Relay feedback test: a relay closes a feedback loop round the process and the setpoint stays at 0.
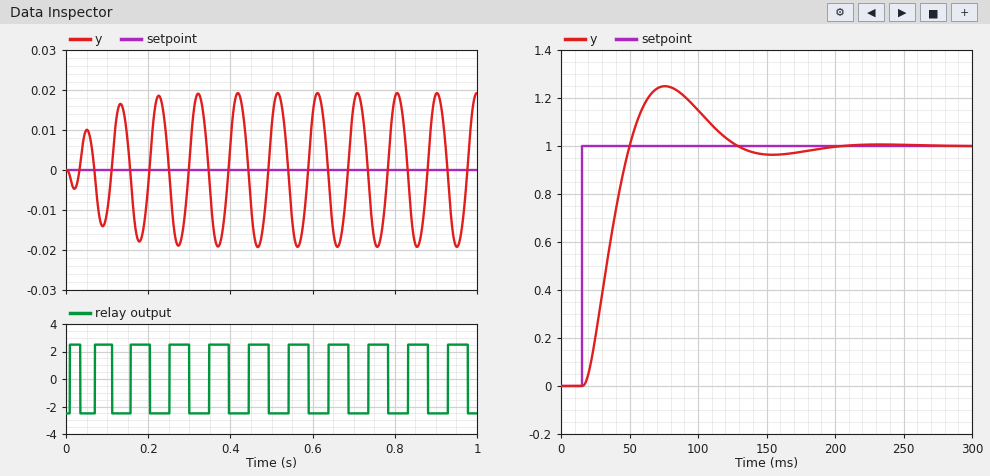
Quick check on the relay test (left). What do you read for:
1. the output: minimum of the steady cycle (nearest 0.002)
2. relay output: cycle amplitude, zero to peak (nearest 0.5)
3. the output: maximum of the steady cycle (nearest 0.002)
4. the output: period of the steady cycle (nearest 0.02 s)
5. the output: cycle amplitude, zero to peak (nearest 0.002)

-0.020
2.5
0.020
0.10 s
0.020
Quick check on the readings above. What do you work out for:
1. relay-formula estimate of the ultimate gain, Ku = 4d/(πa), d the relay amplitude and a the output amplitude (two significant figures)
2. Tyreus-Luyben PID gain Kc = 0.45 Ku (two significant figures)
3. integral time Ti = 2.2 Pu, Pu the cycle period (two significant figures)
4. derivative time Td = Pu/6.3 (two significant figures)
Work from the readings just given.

160
72
0.22 s
0.016 s
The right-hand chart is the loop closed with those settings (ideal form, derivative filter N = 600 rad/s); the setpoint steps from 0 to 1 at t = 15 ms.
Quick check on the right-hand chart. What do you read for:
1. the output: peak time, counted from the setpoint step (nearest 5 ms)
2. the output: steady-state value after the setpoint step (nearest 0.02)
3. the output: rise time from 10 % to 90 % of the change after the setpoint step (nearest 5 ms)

60 ms
1.00
25 ms
